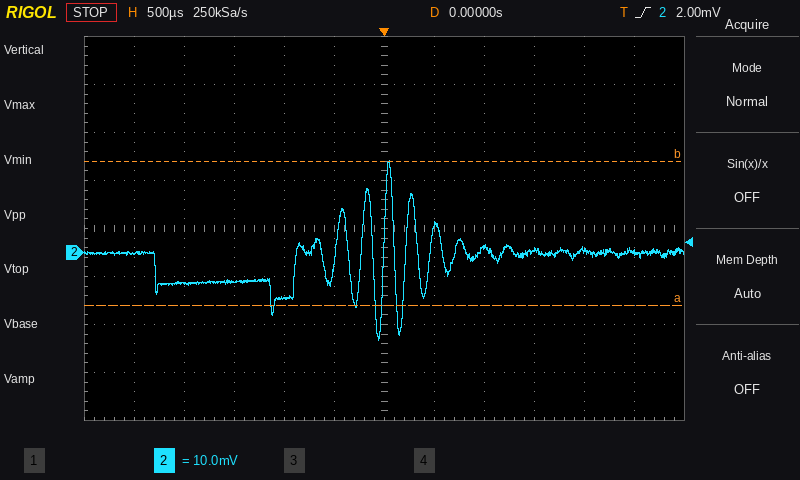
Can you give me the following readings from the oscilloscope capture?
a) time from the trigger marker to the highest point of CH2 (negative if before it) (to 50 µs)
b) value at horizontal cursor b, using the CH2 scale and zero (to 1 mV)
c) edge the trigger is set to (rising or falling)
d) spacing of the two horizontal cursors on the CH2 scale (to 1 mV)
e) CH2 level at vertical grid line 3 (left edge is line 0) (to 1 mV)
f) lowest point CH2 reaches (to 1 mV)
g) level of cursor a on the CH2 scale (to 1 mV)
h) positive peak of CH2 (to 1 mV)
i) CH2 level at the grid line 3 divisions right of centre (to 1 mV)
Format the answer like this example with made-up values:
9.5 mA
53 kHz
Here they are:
+50 µs
19 mV
rising
30 mV
-6 mV
-18 mV
-11 mV
19 mV
0 mV
